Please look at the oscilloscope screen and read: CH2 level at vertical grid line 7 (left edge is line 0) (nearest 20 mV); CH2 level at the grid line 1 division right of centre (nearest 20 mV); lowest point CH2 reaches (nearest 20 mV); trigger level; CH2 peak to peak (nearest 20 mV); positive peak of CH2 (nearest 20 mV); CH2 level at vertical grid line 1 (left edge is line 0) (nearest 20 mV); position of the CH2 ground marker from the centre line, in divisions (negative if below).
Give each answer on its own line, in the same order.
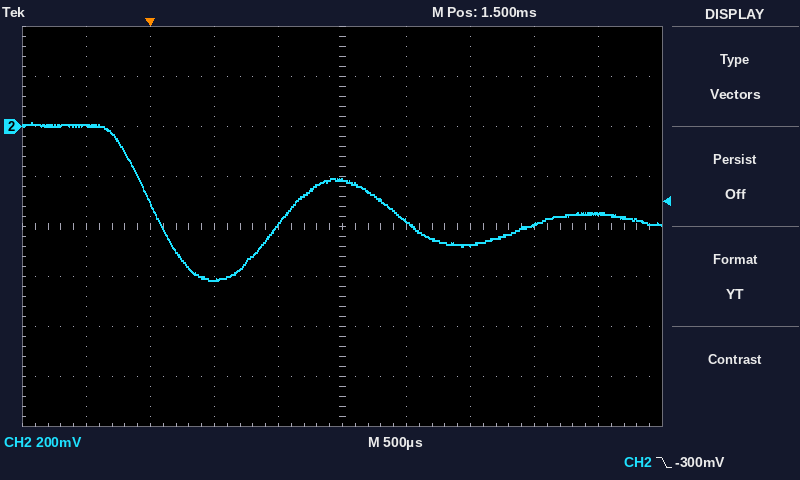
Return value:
-480 mV
-380 mV
-620 mV
-300 mV
640 mV
20 mV
0 mV
+2.0 div
